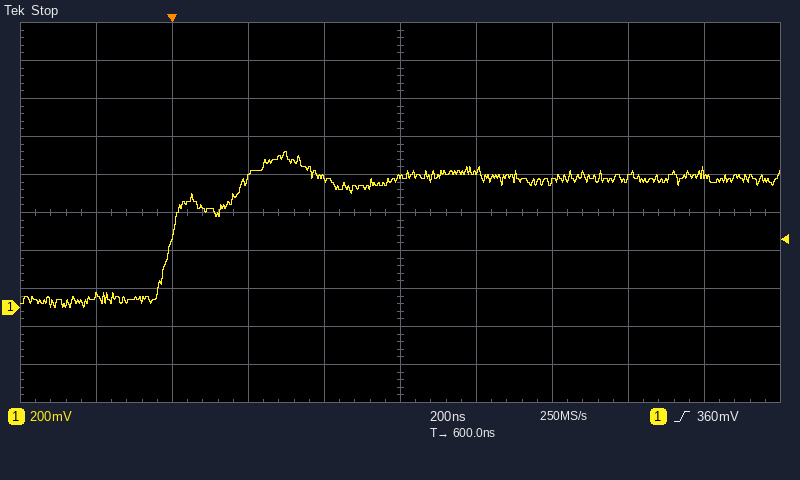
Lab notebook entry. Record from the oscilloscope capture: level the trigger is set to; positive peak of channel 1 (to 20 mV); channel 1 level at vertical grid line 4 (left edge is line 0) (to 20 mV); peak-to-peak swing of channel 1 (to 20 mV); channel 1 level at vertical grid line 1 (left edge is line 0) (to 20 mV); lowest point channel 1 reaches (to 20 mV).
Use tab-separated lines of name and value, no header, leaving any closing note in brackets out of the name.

level the trigger is set to	360 mV
positive peak of channel 1	820 mV
channel 1 level at vertical grid line 4 (left edge is line 0)	680 mV
peak-to-peak swing of channel 1	820 mV
channel 1 level at vertical grid line 1 (left edge is line 0)	60 mV
lowest point channel 1 reaches	0 mV
